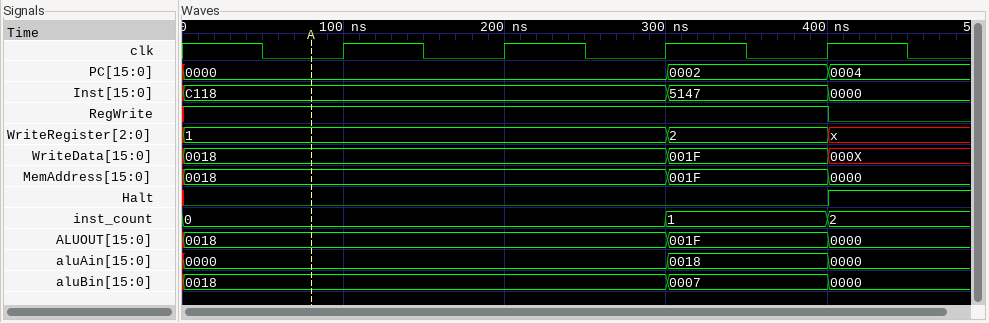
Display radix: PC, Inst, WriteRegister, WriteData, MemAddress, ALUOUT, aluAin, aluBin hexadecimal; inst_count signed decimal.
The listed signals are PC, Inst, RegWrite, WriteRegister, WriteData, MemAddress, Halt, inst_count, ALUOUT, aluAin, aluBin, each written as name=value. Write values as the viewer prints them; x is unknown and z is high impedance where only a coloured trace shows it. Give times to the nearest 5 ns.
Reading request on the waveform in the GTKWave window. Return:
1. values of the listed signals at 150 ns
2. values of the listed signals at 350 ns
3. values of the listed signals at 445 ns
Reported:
PC=0000, Inst=C118, RegWrite=1, WriteRegister=1, WriteData=0018, MemAddress=0018, Halt=0, inst_count=0, ALUOUT=0018, aluAin=0000, aluBin=0018
PC=0002, Inst=5147, RegWrite=1, WriteRegister=2, WriteData=001F, MemAddress=001F, Halt=0, inst_count=1, ALUOUT=001F, aluAin=0018, aluBin=0007
PC=0004, Inst=0000, RegWrite=0, WriteRegister=x, WriteData=000X, MemAddress=0000, Halt=1, inst_count=2, ALUOUT=0000, aluAin=0000, aluBin=0000
